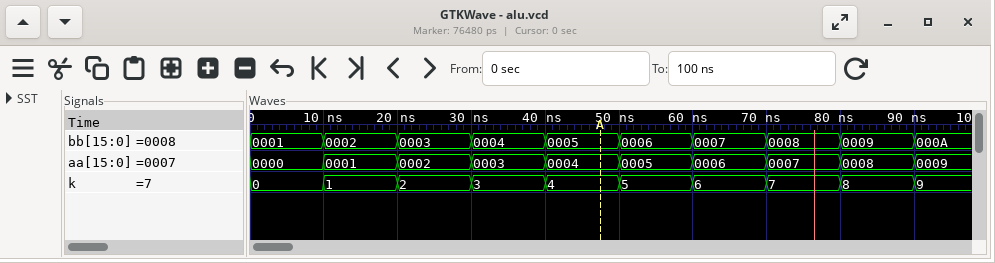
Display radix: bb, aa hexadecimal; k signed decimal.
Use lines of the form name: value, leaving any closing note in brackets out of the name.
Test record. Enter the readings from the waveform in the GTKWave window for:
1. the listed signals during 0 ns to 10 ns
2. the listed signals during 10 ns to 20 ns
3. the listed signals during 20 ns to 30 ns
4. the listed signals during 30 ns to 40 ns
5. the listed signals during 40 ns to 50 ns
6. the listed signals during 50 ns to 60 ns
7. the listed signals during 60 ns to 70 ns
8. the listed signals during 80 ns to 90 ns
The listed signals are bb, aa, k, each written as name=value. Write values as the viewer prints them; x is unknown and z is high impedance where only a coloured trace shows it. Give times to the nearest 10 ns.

the listed signals during 0 ns to 10 ns: bb=0001, aa=0000, k=0
the listed signals during 10 ns to 20 ns: bb=0002, aa=0001, k=1
the listed signals during 20 ns to 30 ns: bb=0003, aa=0002, k=2
the listed signals during 30 ns to 40 ns: bb=0004, aa=0003, k=3
the listed signals during 40 ns to 50 ns: bb=0005, aa=0004, k=4
the listed signals during 50 ns to 60 ns: bb=0006, aa=0005, k=5
the listed signals during 60 ns to 70 ns: bb=0007, aa=0006, k=6
the listed signals during 80 ns to 90 ns: bb=0009, aa=0008, k=8
